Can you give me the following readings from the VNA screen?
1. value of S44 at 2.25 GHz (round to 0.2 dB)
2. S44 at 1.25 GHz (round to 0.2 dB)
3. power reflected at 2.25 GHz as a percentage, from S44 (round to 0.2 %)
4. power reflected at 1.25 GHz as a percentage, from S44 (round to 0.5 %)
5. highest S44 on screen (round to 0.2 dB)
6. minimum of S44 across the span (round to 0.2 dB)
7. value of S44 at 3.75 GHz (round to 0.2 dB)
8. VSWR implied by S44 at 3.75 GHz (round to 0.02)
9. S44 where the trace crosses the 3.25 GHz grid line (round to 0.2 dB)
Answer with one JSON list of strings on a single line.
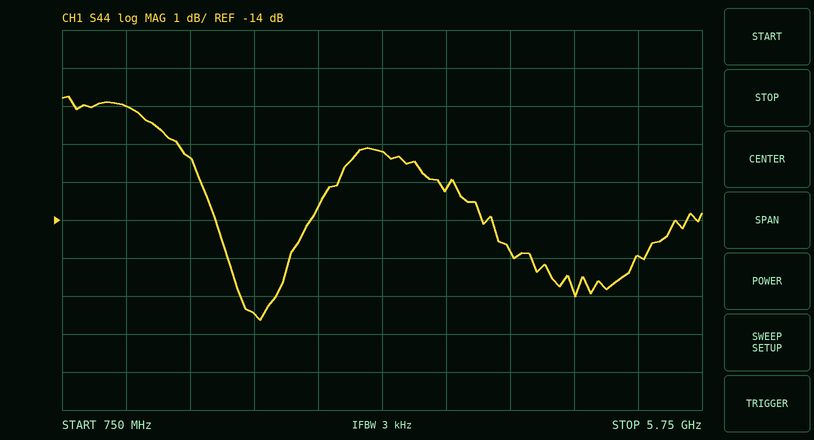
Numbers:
["-16.4 dB", "-11.0 dB", "2.2 %", "8.0 %", "-10.8 dB", "-16.6 dB", "-13.2 dB", "1.56", "-12.2 dB"]
